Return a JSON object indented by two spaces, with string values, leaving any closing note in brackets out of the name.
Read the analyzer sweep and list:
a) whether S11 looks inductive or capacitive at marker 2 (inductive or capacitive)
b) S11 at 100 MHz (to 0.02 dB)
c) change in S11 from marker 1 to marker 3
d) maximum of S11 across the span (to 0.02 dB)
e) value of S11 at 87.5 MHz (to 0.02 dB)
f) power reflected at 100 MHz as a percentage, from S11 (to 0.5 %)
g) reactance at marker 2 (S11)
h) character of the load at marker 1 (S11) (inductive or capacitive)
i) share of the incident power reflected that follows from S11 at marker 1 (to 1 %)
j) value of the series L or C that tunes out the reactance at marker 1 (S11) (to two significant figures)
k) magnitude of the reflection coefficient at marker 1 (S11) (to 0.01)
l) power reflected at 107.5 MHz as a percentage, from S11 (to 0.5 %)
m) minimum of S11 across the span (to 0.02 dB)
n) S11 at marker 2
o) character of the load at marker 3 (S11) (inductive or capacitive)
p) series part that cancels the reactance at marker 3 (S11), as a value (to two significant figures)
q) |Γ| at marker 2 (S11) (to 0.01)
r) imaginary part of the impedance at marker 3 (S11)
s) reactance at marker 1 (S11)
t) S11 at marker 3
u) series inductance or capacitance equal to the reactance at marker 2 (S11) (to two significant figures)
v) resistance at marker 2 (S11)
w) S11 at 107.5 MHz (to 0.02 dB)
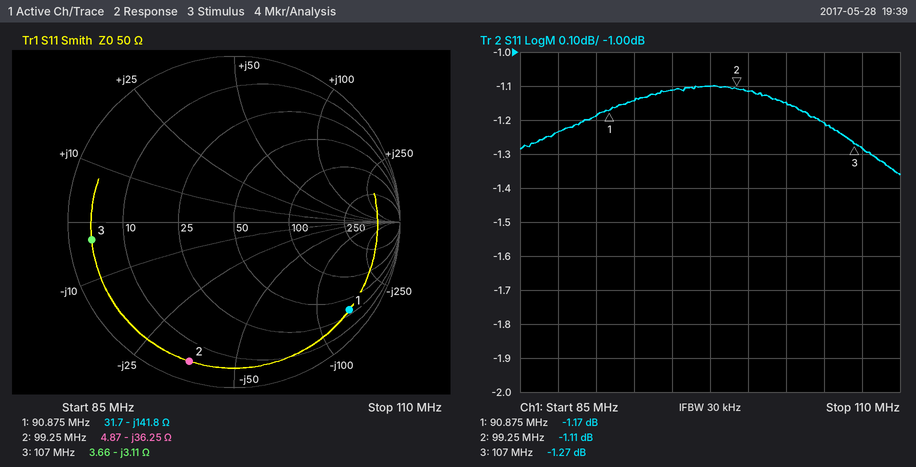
{
  "whether S11 looks inductive or capacitive at marker 2": "capacitive",
  "S11 at 100 MHz": "-1.12 dB",
  "change in S11 from marker 1 to marker 3": "-0.10 dB",
  "maximum of S11 across the span": "-1.10 dB",
  "value of S11 at 87.5 MHz": "-1.24 dB",
  "power reflected at 100 MHz as a percentage, from S11": "77.5 %",
  "reactance at marker 2": "-36.25 Ω",
  "character of the load at marker 1 (S11)": "capacitive",
  "share of the incident power reflected that follows from S11 at marker 1": "76 %",
  "value of the series L or C that tunes out the reactance at marker 1 (S11)": "250 nH",
  "magnitude of the reflection coefficient at marker 1 (S11)": "0.87",
  "power reflected at 107.5 MHz as a percentage, from S11": "74.5 %",
  "minimum of S11 across the span": "-1.36 dB",
  "S11 at marker 2": "-1.11 dB",
  "character of the load at marker 3 (S11)": "capacitive",
  "series part that cancels the reactance at marker 3 (S11), as a value": "4.6 nH",
  "|Γ| at marker 2 (S11)": "0.88",
  "imaginary part of the impedance at marker 3": "-3.11 Ω",
  "reactance at marker 1": "-141.8 Ω",
  "S11 at marker 3": "-1.27 dB",
  "series inductance or capacitance equal to the reactance at marker 2 (S11)": "44 pF",
  "resistance at marker 2": "4.87 Ω",
  "S11 at 107.5 MHz": "-1.28 dB"
}
